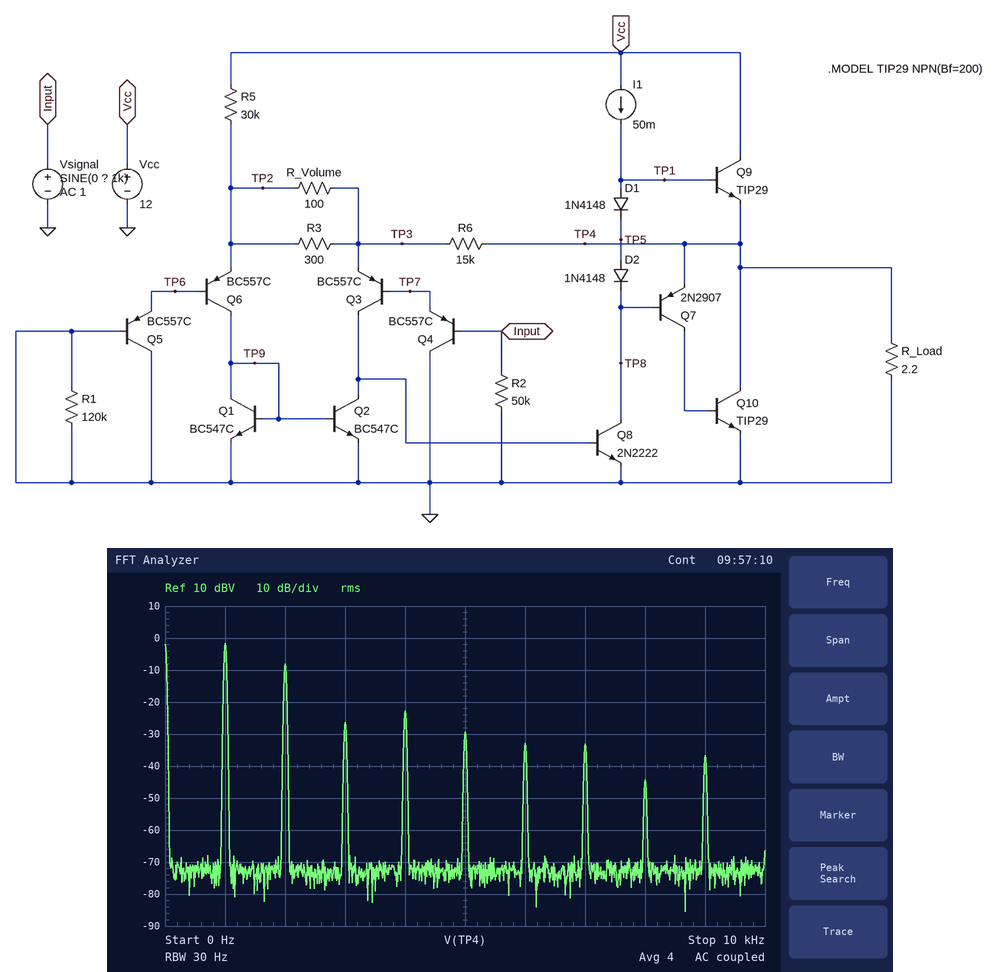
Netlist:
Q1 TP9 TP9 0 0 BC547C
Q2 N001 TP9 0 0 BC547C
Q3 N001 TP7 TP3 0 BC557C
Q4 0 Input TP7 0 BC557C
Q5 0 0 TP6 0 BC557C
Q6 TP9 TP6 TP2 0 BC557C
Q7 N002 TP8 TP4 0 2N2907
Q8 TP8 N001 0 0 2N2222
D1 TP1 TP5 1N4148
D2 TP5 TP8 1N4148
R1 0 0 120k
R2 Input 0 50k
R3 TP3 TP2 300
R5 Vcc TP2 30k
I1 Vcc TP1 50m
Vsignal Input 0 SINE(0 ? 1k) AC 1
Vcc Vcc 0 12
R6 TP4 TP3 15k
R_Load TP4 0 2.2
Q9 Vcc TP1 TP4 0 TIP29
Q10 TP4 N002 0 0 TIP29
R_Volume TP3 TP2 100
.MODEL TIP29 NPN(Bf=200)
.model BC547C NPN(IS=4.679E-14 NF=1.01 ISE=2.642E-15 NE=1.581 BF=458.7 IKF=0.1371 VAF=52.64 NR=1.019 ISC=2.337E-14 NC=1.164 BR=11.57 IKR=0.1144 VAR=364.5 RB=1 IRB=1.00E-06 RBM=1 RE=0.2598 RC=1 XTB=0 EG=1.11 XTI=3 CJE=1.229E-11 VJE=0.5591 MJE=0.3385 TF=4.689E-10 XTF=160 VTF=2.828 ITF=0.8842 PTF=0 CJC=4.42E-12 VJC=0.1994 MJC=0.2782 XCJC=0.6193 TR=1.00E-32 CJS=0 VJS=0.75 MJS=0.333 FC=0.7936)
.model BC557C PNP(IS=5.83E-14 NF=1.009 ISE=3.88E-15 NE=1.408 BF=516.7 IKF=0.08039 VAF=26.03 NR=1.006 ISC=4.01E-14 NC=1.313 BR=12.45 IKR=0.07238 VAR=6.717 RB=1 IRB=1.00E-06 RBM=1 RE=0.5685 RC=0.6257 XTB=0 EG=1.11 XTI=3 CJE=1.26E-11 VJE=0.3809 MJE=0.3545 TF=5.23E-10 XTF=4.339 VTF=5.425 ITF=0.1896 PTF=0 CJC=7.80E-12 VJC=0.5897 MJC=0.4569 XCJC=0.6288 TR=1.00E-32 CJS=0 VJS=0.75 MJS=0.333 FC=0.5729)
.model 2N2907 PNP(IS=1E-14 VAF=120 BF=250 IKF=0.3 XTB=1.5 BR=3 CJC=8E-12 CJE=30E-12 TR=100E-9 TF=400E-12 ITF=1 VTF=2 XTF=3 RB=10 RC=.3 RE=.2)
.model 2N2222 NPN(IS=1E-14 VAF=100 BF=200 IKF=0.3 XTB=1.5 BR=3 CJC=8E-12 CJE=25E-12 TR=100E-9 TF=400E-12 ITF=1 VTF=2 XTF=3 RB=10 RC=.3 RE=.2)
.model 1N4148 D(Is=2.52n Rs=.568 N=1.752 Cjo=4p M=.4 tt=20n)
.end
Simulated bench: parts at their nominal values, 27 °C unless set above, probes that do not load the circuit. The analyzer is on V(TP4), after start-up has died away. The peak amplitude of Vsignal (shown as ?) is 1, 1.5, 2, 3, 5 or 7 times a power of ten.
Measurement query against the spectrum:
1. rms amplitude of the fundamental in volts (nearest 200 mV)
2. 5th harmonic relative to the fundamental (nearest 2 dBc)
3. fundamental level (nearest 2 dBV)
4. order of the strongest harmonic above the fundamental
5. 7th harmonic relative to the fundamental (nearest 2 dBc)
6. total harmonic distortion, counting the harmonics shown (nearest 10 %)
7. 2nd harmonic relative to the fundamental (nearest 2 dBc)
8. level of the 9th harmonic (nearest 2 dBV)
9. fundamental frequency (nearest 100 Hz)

800 mV
-28 dBc
-2 dBV
2
-32 dBc
50 %
-6 dBc
-36 dBV
1.0 kHz
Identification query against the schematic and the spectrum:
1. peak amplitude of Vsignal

15 mV
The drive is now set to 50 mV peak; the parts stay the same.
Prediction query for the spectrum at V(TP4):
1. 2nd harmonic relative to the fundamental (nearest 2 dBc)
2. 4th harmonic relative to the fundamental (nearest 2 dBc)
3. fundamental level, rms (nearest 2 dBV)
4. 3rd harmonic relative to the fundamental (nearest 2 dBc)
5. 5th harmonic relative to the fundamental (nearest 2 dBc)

-8 dBc
-18 dBc
8 dBV
-28 dBc
-48 dBc
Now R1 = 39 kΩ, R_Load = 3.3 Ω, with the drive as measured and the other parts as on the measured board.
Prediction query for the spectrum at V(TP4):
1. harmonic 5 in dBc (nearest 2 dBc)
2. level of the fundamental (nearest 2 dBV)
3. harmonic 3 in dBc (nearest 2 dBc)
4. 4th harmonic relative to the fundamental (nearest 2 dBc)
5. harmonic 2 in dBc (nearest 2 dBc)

-32 dBc
-10 dBV
-8 dBc
-18 dBc
-4 dBc
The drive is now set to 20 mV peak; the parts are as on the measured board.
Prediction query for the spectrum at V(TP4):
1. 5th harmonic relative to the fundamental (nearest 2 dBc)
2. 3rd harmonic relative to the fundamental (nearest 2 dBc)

-30 dBc
-30 dBc
